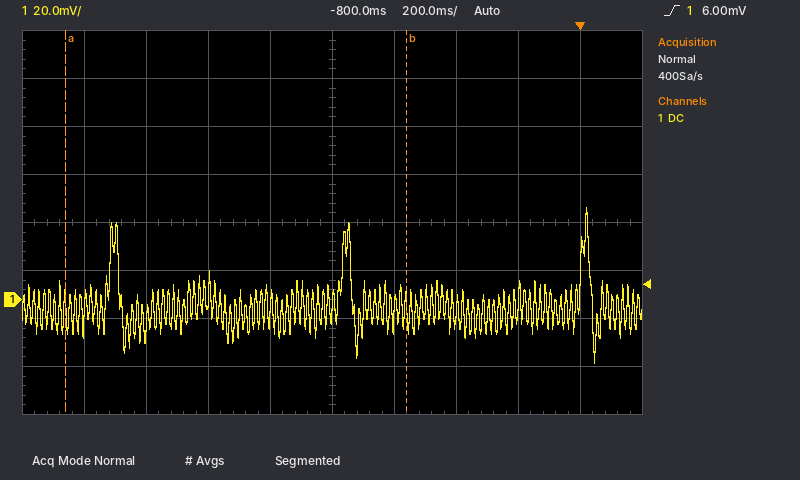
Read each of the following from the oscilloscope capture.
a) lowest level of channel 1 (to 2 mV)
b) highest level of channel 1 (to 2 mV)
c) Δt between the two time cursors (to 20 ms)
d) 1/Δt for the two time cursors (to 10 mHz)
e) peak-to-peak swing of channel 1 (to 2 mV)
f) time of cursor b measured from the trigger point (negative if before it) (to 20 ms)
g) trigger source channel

-26 mV
38 mV
1.10 s
910 mHz
64 mV
-560 ms
channel 1
